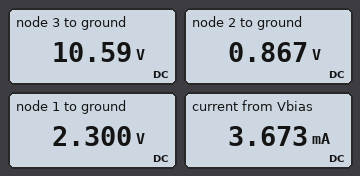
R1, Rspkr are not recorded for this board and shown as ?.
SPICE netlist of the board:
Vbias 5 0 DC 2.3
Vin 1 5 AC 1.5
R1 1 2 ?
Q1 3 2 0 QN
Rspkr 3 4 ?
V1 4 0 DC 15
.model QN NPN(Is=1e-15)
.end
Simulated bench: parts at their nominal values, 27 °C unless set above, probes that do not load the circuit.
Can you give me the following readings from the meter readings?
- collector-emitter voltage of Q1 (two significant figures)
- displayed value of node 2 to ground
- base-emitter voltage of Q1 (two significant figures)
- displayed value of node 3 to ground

11 V
0.867 V
870 mV
10.59 V
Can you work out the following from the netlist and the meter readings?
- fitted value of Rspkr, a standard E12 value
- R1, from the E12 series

12 Ω
390 Ω
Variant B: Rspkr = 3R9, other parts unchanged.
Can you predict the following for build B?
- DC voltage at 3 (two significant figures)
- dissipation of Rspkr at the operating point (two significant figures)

14 V
530 mW
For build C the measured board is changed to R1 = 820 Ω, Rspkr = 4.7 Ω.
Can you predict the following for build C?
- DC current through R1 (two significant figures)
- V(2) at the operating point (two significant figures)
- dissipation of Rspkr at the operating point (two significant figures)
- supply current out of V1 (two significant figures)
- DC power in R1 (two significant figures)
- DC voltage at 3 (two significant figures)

1.8 mA
850 mV
150 mW
180 mA
2.6 mW
14 V
